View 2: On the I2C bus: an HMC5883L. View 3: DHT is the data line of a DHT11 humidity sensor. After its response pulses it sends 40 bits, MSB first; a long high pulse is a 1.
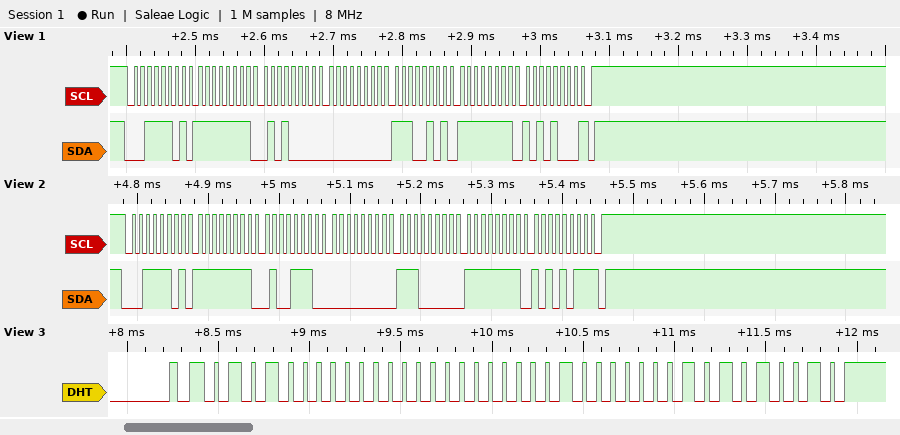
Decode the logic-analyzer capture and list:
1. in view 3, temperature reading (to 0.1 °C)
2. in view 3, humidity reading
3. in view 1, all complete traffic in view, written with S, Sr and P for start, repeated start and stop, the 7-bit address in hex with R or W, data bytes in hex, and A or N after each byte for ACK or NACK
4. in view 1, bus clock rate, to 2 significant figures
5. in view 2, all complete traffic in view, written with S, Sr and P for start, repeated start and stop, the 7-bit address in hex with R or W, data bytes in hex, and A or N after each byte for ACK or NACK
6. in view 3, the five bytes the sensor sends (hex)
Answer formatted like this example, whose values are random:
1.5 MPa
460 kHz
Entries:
1.1 °C
80 %
S 1ER A FF A 50 A 00 A E5 A FF A A8 N P
100 kHz
S 1ER A FF A 4E A 00 A E0 A FF A AB N P
50 00 01 01 52
